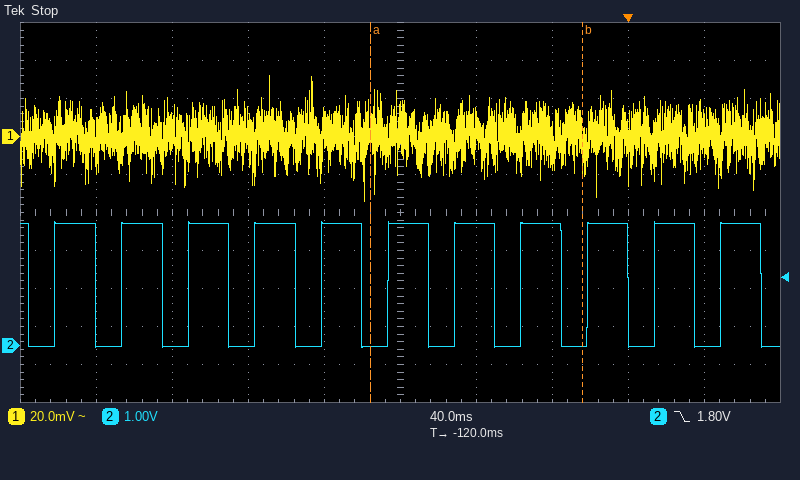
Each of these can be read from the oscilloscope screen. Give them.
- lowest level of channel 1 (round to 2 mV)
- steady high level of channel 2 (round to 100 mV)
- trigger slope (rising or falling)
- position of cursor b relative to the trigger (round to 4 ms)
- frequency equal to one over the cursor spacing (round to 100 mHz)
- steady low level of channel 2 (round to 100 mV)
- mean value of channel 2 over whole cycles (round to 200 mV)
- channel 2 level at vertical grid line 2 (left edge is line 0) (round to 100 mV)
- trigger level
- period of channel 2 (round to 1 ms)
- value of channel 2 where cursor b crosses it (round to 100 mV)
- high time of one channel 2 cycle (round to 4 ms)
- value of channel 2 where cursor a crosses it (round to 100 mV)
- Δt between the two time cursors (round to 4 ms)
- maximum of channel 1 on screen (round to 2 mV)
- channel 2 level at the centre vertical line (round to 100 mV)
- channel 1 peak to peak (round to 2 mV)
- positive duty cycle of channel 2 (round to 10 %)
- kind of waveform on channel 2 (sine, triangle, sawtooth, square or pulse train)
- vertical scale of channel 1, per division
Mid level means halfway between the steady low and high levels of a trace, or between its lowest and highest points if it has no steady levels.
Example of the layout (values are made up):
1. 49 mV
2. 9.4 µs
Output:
1. -34 mV
2. 3.2 V
3. falling
4. -24 ms
5. 8.9 Hz
6. 0.0 V
7. 2.0 V
8. 0.0 V
9. 1.80 V
10. 35 ms
11. 0.0 V
12. 20 ms
13. 0.0 V
14. 112 ms
15. 32 mV
16. 3.2 V
17. 66 mV
18. 60 %
19. pulse train
20. 20 mV
